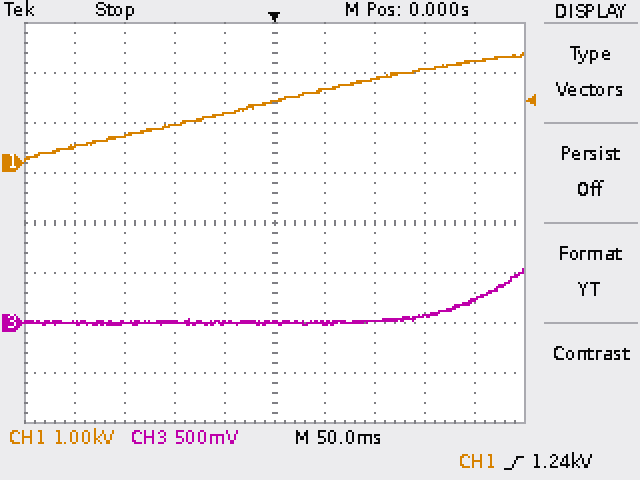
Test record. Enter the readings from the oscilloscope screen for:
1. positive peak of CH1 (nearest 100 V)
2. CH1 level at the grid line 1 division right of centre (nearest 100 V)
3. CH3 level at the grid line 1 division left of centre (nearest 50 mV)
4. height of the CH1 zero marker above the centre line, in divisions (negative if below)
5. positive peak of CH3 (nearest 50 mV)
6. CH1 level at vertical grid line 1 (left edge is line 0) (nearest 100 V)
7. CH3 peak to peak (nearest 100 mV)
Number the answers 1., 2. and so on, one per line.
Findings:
1. 2.2 kV
2. 1.5 kV
3. 0 mV
4. +1.2 div
5. 550 mV
6. 300 V
7. 600 mV
